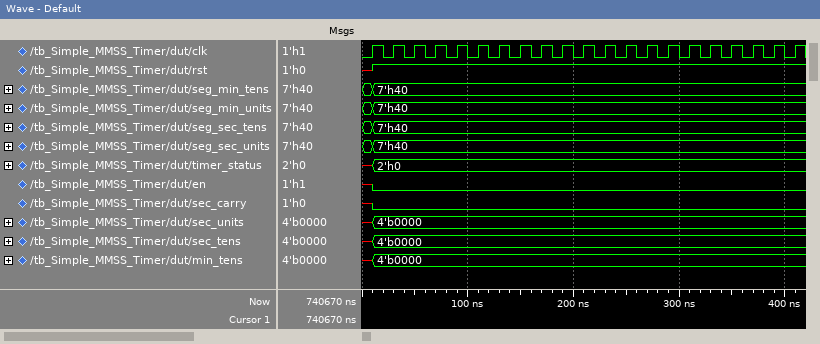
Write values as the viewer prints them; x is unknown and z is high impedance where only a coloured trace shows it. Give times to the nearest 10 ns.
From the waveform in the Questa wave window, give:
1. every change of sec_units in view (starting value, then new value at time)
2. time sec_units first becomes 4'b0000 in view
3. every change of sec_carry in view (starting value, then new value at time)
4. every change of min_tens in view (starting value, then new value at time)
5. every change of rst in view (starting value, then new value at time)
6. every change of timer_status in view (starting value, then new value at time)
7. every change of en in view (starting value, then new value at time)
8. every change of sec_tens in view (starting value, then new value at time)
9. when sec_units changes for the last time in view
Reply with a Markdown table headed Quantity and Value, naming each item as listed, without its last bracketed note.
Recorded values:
| Quantity | Value |
|---|---|
| every change of sec_units in view | x, 4'b0000 at 10 ns |
| time sec_units first becomes 4'b0000 in view | 10 ns |
| every change of sec_carry in view | x, 0 at 10 ns |
| every change of min_tens in view | x, 4'b0000 at 10 ns |
| every change of rst in view | x, 1 at 10 ns |
| every change of timer_status in view | x, 2'h0 at 10 ns |
| every change of en in view | x, 0 at 10 ns |
| every change of sec_tens in view | x, 4'b0000 at 10 ns |
| when sec_units changes for the last time in view | 10 ns |
